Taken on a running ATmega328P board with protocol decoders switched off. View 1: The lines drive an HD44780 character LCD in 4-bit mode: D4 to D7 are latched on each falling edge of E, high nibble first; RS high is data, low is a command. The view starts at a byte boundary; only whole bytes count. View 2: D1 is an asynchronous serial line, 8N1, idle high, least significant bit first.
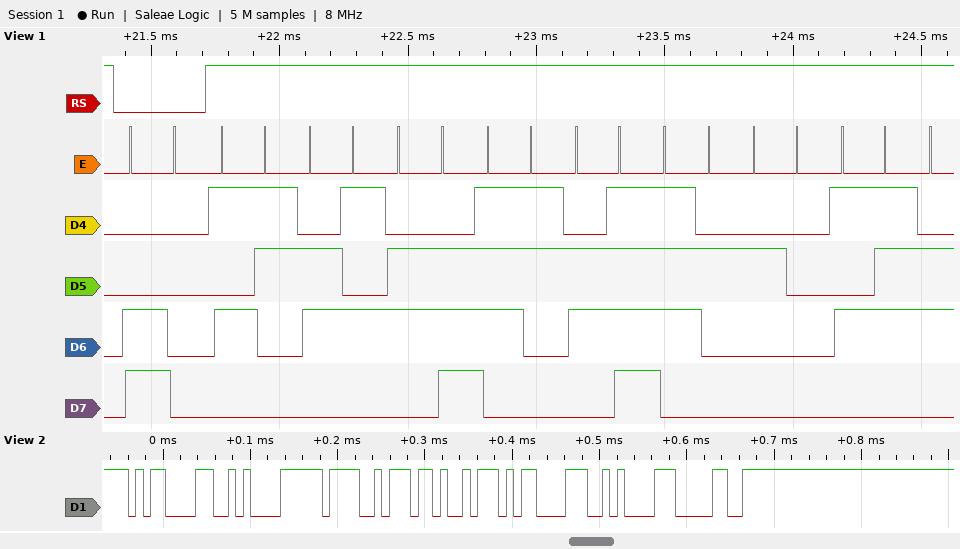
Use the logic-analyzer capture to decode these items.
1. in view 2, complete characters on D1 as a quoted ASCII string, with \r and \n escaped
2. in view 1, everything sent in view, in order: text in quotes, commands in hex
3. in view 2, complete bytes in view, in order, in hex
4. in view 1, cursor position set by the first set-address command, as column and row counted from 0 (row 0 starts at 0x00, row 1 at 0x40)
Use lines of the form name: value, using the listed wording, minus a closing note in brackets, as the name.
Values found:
in view 2, complete characters on D1 as a quoted ASCII string, with \r and \n escaped: "\r\nOK\r\n0"
in view 1, everything sent in view, in order: text in quotes, commands in hex: 0xC0 "Sensor W"
in view 2, complete bytes in view, in order, in hex: 0D 0A 4F 4B 0D 0A 30
in view 1, cursor position set by the first set-address command, as column and row counted from 0: column 0, row 1
